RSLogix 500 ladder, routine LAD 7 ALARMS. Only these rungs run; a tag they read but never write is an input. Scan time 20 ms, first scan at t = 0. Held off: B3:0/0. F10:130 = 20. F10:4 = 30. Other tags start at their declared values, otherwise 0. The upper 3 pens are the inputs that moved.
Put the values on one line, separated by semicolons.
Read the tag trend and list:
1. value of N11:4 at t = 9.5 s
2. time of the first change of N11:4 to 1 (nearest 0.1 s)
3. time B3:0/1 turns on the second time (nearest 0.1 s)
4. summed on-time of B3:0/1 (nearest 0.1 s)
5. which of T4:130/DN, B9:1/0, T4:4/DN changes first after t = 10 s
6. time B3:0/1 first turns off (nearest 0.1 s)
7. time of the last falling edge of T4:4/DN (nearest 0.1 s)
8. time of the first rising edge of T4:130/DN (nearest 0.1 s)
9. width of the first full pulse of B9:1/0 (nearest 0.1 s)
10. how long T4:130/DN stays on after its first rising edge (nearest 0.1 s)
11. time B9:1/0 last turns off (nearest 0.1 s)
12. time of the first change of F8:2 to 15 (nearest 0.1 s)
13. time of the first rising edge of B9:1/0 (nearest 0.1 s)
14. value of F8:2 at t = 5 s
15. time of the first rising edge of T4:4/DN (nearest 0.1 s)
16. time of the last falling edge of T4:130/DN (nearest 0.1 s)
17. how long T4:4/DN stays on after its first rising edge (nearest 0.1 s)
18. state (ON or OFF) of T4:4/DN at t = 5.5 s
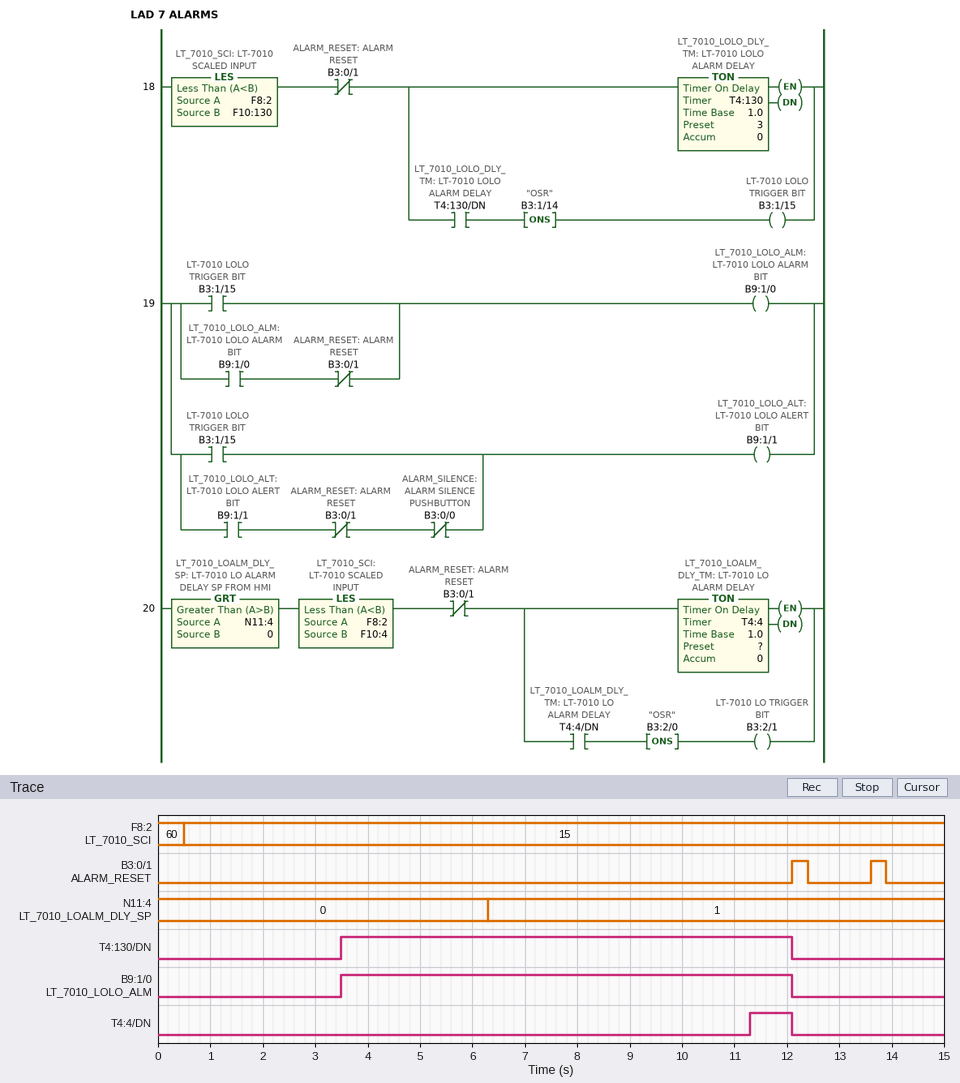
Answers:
1; 6.3 s; 13.6 s; 0.6 s; T4:4/DN; 12.4 s; 12.1 s; 3.5 s; 8.6 s; 8.6 s; 12.1 s; 0.5 s; 3.5 s; 15; 11.3 s; 12.1 s; 0.8 s; OFF
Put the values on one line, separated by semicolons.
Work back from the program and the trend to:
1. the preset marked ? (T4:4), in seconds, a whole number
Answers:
5 s
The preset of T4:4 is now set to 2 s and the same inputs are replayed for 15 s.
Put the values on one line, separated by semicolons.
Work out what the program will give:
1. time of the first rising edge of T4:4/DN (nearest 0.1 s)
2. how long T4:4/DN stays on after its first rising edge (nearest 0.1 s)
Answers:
8.3 s; 3.8 s
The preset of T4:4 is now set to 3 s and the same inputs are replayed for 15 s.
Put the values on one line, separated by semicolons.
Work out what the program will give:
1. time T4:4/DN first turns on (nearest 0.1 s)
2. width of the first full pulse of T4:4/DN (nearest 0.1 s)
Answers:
9.3 s; 2.8 s
